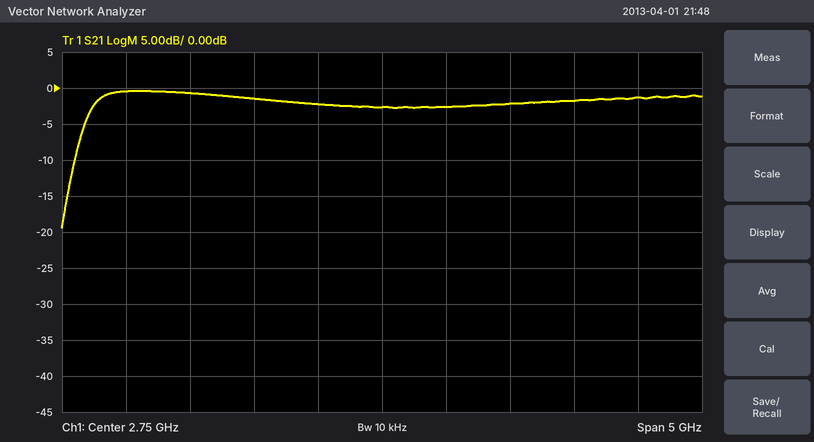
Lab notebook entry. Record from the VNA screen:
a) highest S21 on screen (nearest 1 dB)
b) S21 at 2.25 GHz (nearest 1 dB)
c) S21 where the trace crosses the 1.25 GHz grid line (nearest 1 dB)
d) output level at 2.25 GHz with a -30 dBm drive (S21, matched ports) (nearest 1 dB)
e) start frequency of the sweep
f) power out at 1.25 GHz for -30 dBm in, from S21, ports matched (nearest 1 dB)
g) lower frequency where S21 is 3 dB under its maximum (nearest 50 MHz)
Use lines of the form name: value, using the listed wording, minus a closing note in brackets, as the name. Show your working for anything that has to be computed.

highest S21 on screen: 0 dB
S21 at 2.25 GHz: -2 dB
S21 where the trace crosses the 1.25 GHz grid line: -1 dB
output level at 2.25 GHz with a -30 dBm drive (S21, matched ports): -30 dBm + (-2 dB) = -32 dBm
start frequency of the sweep: 250 MHz
power out at 1.25 GHz for -30 dBm in, from S21, ports matched: -30 dBm + (-1 dB) = -31 dBm
lower frequency where S21 is 3 dB under its maximum: 450 MHz
